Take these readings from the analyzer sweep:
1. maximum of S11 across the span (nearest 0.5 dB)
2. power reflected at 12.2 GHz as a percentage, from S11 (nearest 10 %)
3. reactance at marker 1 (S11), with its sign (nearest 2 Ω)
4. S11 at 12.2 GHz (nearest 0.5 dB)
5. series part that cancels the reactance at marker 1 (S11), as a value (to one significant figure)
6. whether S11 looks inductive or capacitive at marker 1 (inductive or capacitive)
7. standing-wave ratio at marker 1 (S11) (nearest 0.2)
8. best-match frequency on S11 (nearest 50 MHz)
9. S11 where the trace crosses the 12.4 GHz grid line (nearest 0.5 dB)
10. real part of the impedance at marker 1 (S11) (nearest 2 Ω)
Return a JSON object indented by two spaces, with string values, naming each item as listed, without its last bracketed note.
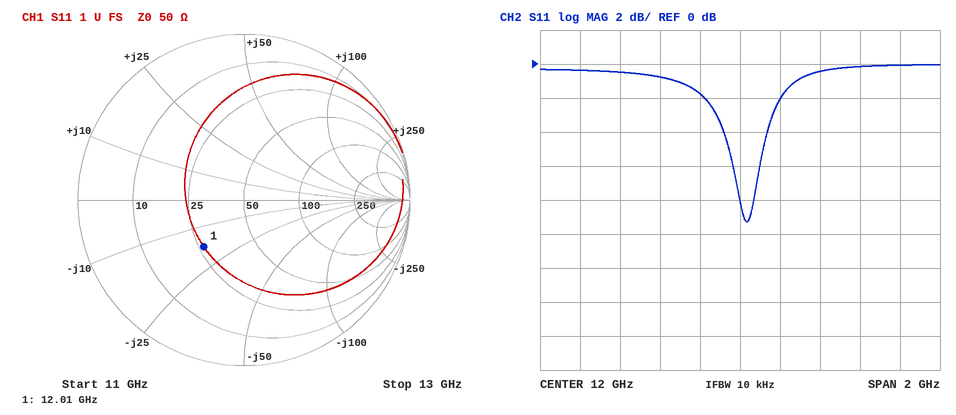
{
  "maximum of S11 across the span": "0.0 dB",
  "power reflected at 12.2 GHz as a percentage, from S11": "60 %",
  "reactance at marker 1 (S11), with its sign": "-18 Ω",
  "S11 at 12.2 GHz": "-2.0 dB",
  "series part that cancels the reactance at marker 1 (S11), as a value": "200 pH",
  "whether S11 looks inductive or capacitive at marker 1": "capacitive",
  "standing-wave ratio at marker 1 (S11)": "2.2",
  "best-match frequency on S11": "12.05 GHz",
  "S11 where the trace crosses the 12.4 GHz grid line": "-0.5 dB",
  "real part of the impedance at marker 1 (S11)": "26 Ω"
}
